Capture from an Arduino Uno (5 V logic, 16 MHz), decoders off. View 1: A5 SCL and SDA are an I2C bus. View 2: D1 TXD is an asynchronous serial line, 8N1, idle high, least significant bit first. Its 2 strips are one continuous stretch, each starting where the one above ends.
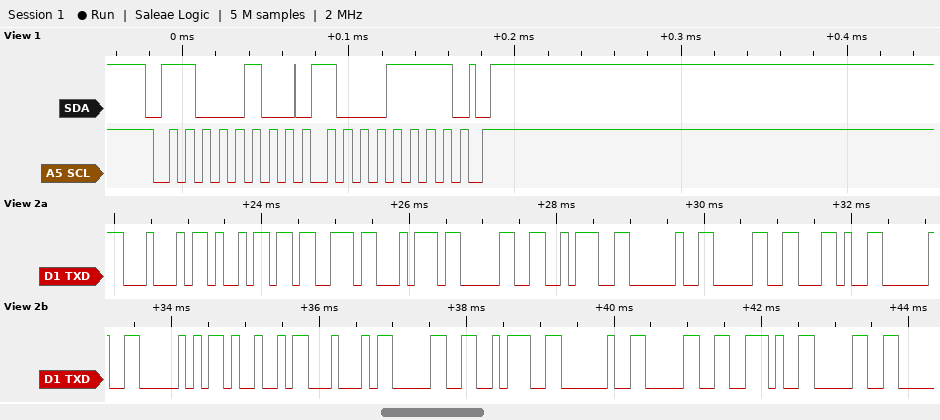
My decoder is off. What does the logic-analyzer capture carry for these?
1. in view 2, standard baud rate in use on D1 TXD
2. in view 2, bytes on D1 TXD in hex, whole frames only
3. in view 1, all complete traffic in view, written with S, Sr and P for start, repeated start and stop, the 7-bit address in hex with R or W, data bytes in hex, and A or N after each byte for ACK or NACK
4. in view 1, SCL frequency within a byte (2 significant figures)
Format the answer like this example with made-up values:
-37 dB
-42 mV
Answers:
9600 baud
44 69 73 74 30 3A 20 30 2C 20 50 49 44 30 3A 20 30 2E 30
S 62W A 8F A P
100 kHz
